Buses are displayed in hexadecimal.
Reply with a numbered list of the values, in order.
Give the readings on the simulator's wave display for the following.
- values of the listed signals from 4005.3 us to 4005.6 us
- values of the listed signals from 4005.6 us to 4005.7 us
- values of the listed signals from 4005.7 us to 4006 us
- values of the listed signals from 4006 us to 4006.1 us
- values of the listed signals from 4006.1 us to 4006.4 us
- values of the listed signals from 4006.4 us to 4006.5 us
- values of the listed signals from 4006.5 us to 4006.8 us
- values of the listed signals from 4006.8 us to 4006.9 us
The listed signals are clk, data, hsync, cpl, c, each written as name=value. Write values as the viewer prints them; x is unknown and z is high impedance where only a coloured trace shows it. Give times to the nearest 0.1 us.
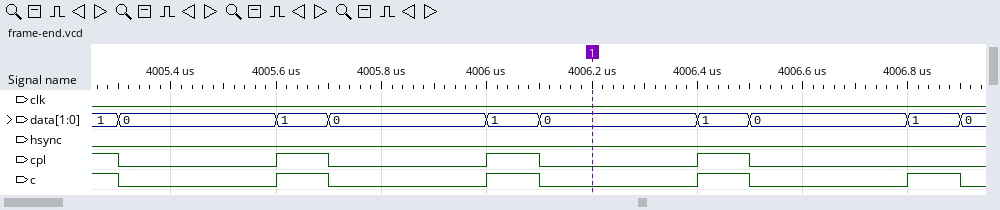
1. clk=0, data=0, hsync=0, cpl=0, c=0
2. clk=0, data=1, hsync=0, cpl=1, c=1
3. clk=0, data=0, hsync=0, cpl=0, c=0
4. clk=0, data=1, hsync=0, cpl=1, c=1
5. clk=0, data=0, hsync=0, cpl=0, c=0
6. clk=0, data=1, hsync=0, cpl=1, c=1
7. clk=0, data=0, hsync=0, cpl=0, c=0
8. clk=0, data=1, hsync=0, cpl=0, c=1
